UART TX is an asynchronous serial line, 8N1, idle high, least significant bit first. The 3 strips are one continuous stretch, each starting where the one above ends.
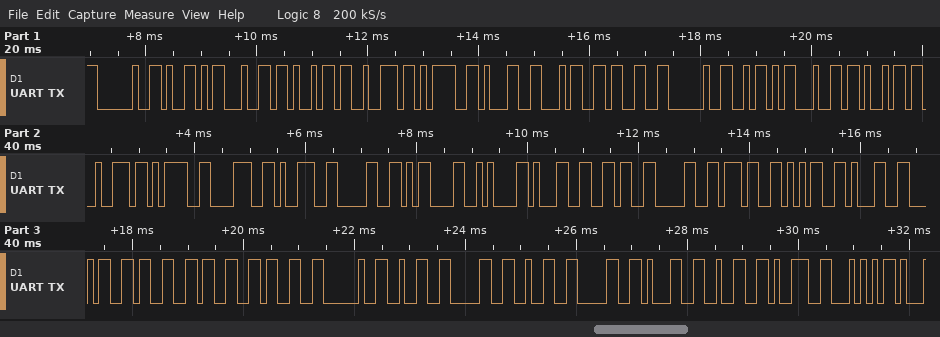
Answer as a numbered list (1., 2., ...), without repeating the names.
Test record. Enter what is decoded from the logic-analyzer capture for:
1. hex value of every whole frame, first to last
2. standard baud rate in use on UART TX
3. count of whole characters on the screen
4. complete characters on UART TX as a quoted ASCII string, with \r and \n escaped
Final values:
1. 20 59 64 69 72 3D 31 34 33 20 5A 64 69 72 3D 38 39 30 0D 0A 31 36 30 37 35 31 34 33 33 33 20 32 30 32 30 31 32 39 54
2. 9600 baud
3. 39
4. " Ydir=143 Zdir=890\r\n1607514333 2020129T"
